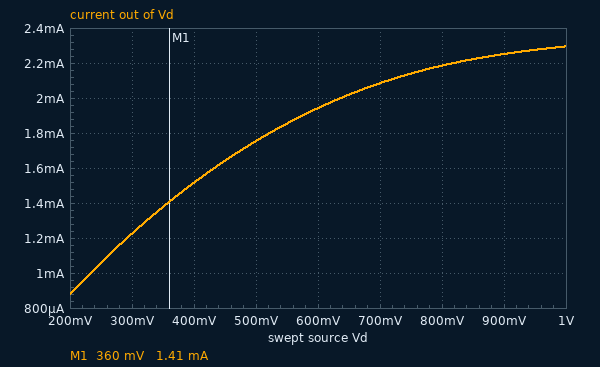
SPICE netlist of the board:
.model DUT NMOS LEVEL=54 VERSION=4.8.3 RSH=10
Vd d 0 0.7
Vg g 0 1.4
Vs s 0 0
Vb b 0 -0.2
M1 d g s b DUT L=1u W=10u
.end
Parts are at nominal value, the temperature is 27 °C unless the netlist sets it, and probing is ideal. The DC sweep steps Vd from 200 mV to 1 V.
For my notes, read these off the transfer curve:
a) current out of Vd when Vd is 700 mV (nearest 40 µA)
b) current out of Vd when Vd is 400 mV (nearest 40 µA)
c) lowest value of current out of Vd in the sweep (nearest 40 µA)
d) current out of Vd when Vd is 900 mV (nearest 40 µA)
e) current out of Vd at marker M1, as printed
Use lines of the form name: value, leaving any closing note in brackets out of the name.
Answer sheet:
current out of Vd when Vd is 700 mV: 2.08 mA
current out of Vd when Vd is 400 mV: 1.52 mA
lowest value of current out of Vd in the sweep: 880 µA
current out of Vd when Vd is 900 mV: 2.24 mA
current out of Vd at marker M1, as printed: 1.41 mA
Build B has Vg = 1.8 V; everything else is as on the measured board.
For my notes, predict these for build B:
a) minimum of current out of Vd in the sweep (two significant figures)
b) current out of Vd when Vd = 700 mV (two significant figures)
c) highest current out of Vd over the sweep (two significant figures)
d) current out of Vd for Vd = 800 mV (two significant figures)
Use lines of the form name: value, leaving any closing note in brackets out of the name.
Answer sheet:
minimum of current out of Vd in the sweep: 1.1 mA
current out of Vd when Vd = 700 mV: 2.9 mA
highest current out of Vd over the sweep: 3.4 mA
current out of Vd for Vd = 800 mV: 3.1 mA
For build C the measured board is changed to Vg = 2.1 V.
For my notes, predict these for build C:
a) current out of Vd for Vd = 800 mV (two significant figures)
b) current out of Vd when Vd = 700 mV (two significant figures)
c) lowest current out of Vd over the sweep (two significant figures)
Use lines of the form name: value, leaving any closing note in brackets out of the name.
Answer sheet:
current out of Vd for Vd = 800 mV: 3.7 mA
current out of Vd when Vd = 700 mV: 3.4 mA
lowest current out of Vd over the sweep: 1.3 mA
